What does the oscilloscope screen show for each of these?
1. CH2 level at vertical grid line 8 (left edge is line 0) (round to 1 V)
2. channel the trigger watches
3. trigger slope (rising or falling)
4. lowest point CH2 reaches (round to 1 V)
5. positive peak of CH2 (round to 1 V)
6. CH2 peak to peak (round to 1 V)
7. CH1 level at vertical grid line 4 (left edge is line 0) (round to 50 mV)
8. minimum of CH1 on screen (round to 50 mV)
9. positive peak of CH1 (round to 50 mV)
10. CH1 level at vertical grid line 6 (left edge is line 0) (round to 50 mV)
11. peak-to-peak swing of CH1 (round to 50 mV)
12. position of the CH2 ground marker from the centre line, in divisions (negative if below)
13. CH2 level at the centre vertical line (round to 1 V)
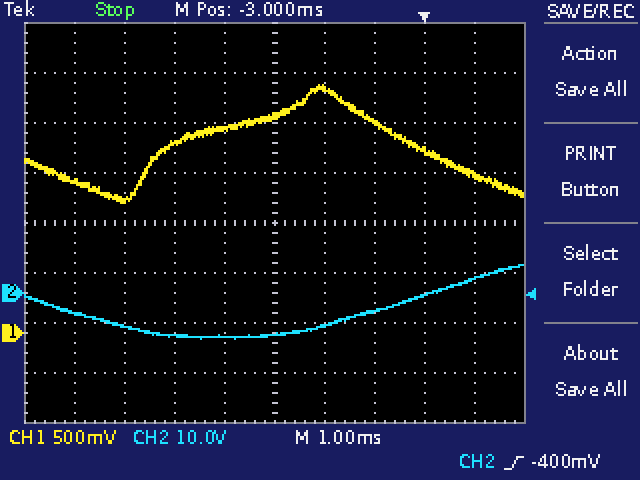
0 V
CH2
rising
-9 V
6 V
15 V
2.05 V
1.30 V
2.50 V
2.45 V
1.20 V
-1.4 div
-8 V
